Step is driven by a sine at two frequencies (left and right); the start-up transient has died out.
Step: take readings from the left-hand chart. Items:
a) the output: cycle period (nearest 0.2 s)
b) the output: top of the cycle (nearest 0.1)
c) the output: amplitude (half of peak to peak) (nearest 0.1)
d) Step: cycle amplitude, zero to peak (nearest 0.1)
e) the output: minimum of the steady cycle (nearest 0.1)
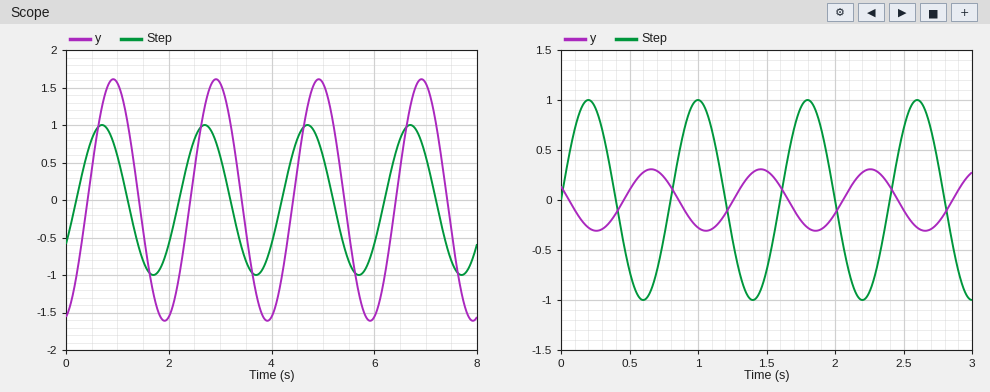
2.0 s
1.6
1.6
1.0
-1.6
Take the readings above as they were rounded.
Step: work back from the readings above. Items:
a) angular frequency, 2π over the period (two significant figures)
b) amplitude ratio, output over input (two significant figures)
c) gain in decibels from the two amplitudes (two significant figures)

3.1 rad/s
1.6
4.1 dB
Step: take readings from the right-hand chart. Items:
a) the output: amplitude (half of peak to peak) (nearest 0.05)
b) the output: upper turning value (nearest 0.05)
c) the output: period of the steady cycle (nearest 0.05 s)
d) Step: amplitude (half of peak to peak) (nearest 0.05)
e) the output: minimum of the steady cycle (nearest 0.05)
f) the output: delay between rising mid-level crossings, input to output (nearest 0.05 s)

0.30
0.30
0.80 s
1.00
-0.30
0.45 s
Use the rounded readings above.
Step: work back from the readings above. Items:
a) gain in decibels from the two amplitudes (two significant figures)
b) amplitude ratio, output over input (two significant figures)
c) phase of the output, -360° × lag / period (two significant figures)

-10 dB
0.30
-200°
